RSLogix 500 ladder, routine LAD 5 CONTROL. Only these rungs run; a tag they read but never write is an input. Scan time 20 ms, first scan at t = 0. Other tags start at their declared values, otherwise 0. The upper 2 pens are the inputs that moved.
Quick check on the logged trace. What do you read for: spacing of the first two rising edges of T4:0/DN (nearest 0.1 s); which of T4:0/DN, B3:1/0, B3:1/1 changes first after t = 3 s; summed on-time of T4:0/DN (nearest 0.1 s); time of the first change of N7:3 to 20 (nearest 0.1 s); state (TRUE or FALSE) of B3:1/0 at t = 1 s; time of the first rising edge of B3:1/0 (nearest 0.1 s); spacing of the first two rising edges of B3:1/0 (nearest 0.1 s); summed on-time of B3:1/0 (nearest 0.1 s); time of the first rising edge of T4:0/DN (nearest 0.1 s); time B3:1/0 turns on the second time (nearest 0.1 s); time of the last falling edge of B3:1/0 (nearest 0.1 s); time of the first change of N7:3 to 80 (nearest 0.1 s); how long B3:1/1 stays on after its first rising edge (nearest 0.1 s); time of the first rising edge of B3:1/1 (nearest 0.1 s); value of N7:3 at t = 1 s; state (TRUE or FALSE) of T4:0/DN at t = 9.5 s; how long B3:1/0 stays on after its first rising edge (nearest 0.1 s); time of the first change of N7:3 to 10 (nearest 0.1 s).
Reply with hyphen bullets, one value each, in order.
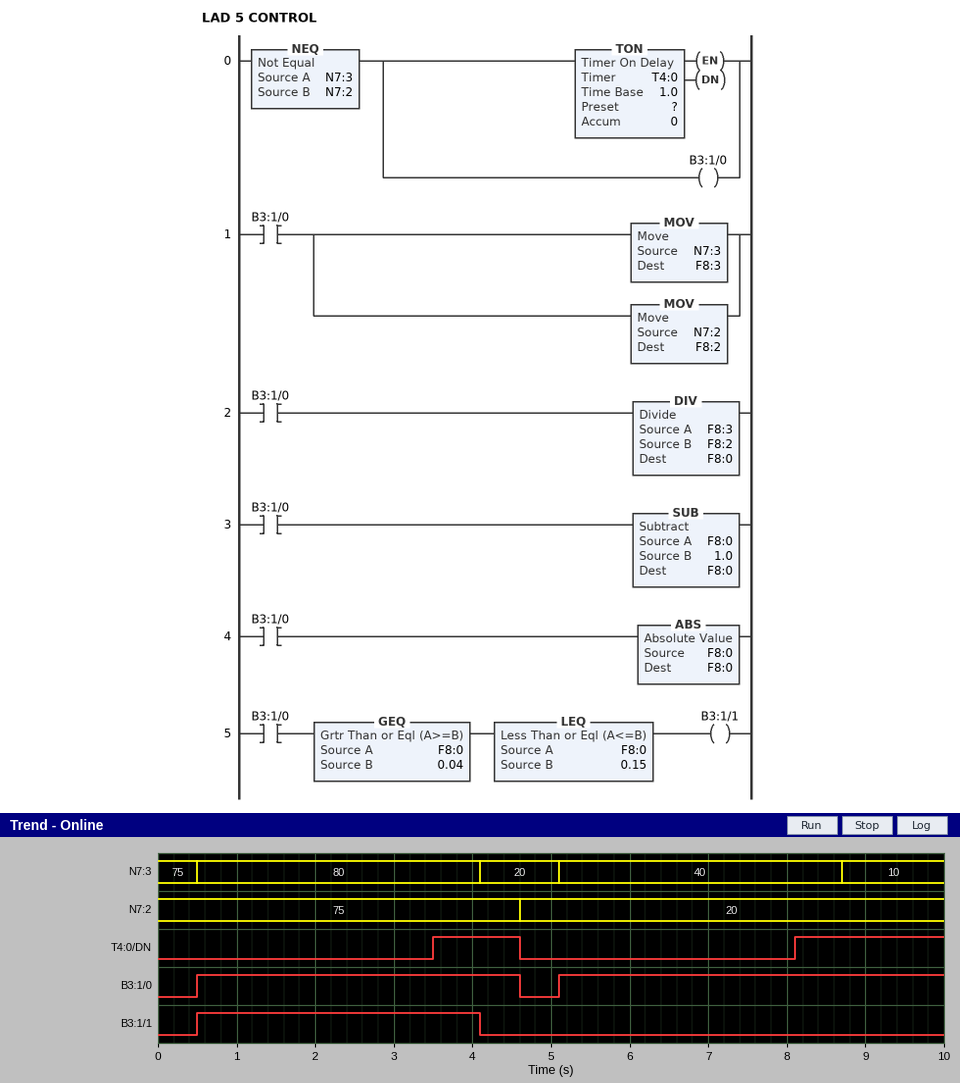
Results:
- 4.6 s
- T4:0/DN
- 3.0 s
- 4.1 s
- TRUE
- 0.5 s
- 4.6 s
- 9.0 s
- 3.5 s
- 5.1 s
- 4.6 s
- 0.5 s
- 3.6 s
- 0.5 s
- 80
- TRUE
- 4.1 s
- 8.7 s
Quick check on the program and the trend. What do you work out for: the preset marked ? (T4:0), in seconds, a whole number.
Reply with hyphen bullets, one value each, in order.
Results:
- 3 s
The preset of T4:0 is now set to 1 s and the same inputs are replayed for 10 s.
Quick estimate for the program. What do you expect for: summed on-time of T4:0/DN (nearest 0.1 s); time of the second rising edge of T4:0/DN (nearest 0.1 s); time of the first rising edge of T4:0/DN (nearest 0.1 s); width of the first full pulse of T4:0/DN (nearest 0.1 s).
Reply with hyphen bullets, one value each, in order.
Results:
- 7.0 s
- 6.1 s
- 1.5 s
- 3.1 s
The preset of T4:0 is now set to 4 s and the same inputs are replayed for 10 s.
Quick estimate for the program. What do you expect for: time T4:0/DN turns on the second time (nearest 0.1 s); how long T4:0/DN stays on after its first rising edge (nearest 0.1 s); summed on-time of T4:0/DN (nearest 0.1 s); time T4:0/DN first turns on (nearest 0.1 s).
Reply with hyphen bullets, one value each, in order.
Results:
- 9.1 s
- 0.1 s
- 1.0 s
- 4.5 s
